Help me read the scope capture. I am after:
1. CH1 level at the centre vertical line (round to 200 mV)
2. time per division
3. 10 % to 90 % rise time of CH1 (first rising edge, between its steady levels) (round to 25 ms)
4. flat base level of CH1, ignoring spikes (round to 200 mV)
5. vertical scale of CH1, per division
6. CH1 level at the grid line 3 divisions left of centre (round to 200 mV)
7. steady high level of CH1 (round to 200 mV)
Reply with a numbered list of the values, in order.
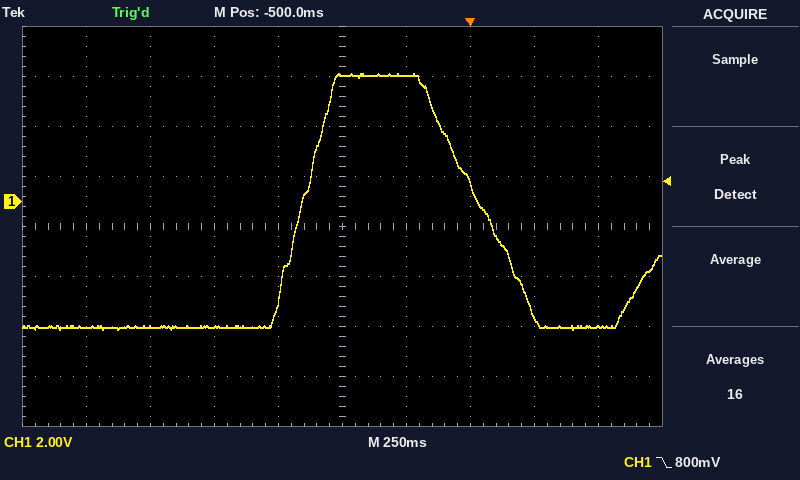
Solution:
1. 5.0 V
2. 250 ms
3. 200 ms
4. -5.0 V
5. 2 V
6. -5.0 V
7. 5.0 V
